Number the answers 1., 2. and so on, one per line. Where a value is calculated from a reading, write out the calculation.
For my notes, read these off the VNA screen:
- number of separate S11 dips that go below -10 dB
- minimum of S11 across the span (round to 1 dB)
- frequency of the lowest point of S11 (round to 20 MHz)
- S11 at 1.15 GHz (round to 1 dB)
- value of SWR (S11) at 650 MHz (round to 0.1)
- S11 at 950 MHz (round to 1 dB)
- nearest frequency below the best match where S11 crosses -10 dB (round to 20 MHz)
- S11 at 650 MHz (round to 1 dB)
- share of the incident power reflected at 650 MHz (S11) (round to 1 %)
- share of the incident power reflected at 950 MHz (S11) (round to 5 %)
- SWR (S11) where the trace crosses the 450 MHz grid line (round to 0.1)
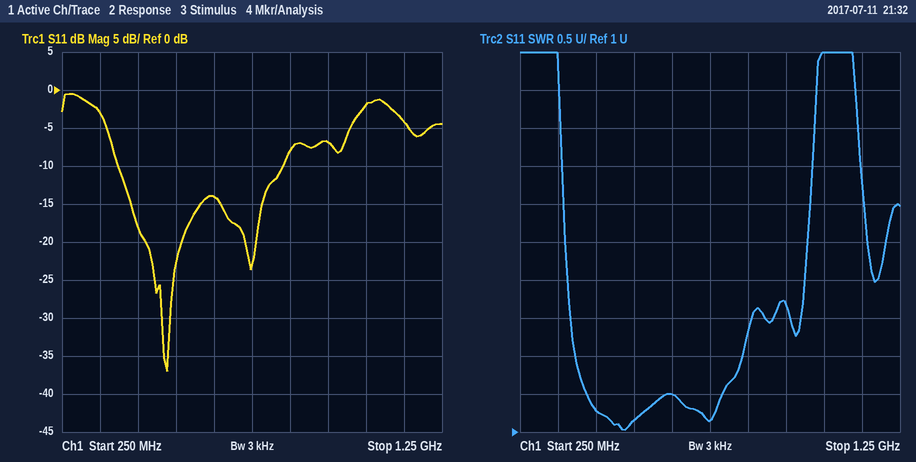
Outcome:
1. 2
2. -37 dB
3. 520 MHz
4. -4 dB
5. 1.5
6. -7 dB
7. 400 MHz
8. -14 dB
9. 10^(-14/10) ≈ 4 %
10. 10^(-7/10) ≈ 20 %
11. 1.3
